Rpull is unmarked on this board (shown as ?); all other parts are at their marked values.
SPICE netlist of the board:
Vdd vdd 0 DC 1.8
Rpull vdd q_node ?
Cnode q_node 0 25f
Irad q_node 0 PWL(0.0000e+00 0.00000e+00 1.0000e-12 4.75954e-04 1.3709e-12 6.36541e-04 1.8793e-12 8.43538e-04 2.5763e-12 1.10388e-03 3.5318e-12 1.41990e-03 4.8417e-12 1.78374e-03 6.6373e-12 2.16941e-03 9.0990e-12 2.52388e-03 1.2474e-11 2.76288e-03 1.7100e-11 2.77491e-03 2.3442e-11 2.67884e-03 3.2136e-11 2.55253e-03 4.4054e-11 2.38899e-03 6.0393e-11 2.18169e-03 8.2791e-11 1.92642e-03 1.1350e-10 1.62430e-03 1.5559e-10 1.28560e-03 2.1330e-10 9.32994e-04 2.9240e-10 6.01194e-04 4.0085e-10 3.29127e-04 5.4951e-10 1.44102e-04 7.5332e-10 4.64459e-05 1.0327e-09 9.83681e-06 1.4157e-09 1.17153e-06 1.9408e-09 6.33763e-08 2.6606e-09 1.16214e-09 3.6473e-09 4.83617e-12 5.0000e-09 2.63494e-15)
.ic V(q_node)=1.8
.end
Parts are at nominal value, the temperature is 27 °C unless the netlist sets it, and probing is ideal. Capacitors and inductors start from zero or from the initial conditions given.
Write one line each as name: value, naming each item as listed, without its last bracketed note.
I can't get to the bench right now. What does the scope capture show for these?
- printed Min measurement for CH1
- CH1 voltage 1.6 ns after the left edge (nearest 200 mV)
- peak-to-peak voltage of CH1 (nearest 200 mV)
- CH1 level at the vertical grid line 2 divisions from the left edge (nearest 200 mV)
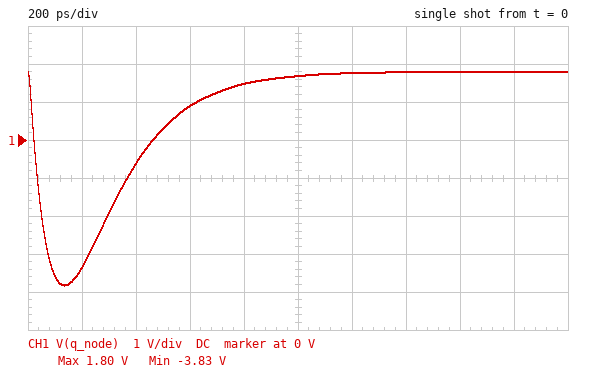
printed Min measurement for CH1: -3.83 V
CH1 voltage 1.6 ns after the left edge: 1.8 V
peak-to-peak voltage of CH1: 5.6 V
CH1 level at the vertical grid line 2 divisions from the left edge: -600 mV
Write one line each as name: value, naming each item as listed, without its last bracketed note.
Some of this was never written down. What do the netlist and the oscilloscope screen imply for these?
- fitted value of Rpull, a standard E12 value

fitted value of Rpull, a standard E12 value: 3.9 kΩ
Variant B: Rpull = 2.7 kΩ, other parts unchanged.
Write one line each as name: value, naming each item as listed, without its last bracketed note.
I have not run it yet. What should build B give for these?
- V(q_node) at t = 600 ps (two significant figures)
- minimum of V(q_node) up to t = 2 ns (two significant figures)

V(q_node) at t = 600 ps: 1.3 V
minimum of V(q_node) up to t = 2 ns: -2.7 V
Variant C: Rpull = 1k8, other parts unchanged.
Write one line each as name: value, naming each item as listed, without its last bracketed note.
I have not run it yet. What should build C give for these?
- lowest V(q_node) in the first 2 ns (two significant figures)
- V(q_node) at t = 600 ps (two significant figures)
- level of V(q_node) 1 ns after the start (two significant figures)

lowest V(q_node) in the first 2 ns: -1.6 V
V(q_node) at t = 600 ps: 1.5 V
level of V(q_node) 1 ns after the start: 1.8 V
